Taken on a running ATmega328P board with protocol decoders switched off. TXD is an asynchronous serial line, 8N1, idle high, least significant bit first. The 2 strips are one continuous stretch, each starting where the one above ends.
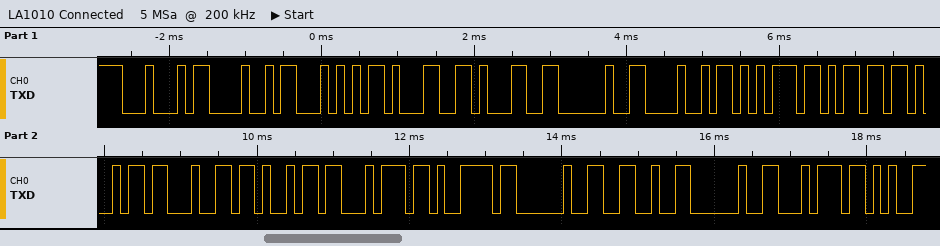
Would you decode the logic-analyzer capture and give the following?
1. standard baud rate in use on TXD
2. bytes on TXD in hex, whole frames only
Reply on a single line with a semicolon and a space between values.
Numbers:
9600 baud; 0x44 0x48 0x54 0x31 0x31 0x20 0x48 0x75 0x6D 0x69 0x64 0x69 0x74 0x79 0x20 0x26 0x20 0x74
